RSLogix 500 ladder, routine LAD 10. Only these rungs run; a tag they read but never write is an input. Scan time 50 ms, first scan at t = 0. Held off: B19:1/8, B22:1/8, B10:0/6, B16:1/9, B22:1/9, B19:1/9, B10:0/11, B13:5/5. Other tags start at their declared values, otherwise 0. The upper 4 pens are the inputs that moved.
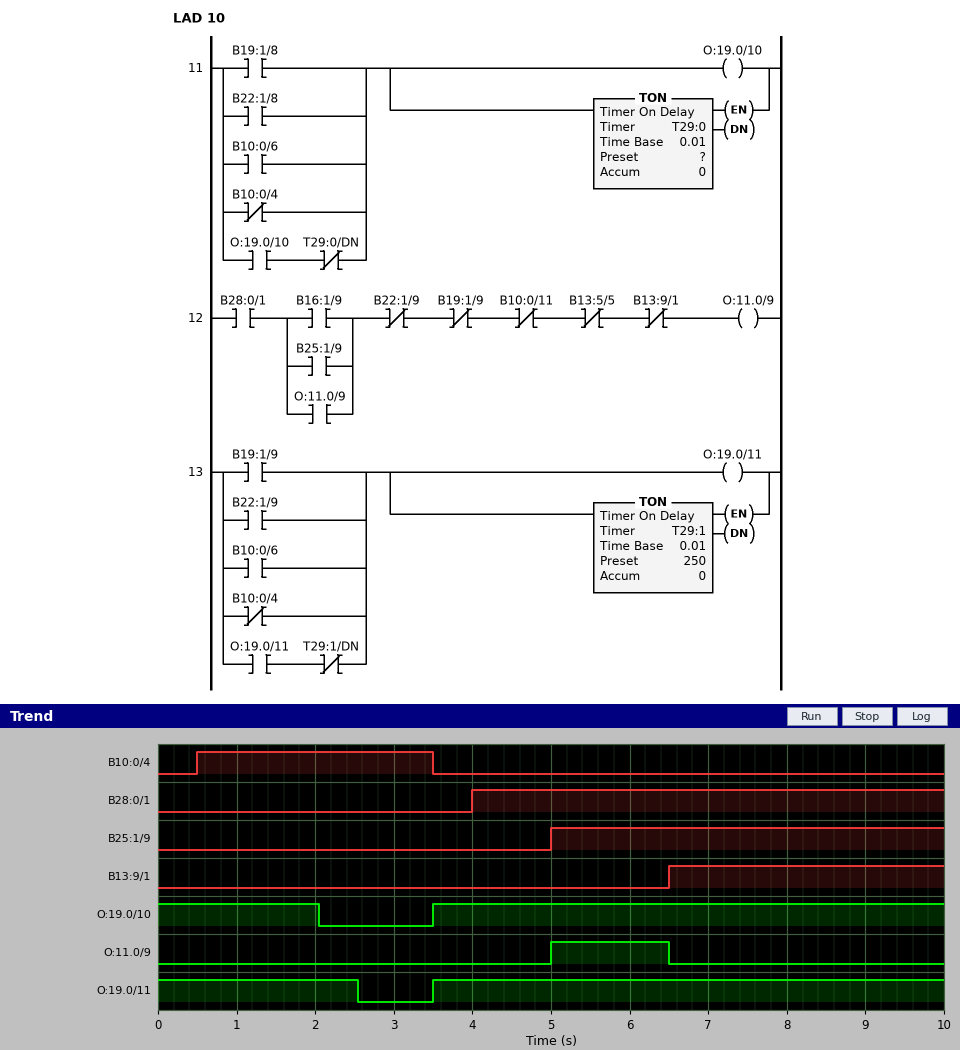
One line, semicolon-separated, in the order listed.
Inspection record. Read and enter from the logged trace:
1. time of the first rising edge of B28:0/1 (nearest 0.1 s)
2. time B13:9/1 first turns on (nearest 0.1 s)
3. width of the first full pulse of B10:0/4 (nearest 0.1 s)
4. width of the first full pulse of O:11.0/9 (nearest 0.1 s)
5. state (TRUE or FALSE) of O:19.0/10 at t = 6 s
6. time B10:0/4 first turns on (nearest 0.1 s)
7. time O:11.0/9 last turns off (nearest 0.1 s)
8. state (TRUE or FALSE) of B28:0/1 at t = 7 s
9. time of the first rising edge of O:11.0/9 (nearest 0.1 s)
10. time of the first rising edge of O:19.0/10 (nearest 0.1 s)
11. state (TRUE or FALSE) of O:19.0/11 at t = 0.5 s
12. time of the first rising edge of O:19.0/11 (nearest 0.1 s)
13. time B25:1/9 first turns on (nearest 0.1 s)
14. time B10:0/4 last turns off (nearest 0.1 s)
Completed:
4.0 s; 6.5 s; 3.0 s; 1.5 s; TRUE; 0.5 s; 6.5 s; TRUE; 5.0 s; 3.5 s; TRUE; 3.5 s; 5.0 s; 3.5 s
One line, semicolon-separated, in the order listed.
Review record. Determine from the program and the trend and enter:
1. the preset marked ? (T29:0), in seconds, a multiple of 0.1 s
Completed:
2.0 s
